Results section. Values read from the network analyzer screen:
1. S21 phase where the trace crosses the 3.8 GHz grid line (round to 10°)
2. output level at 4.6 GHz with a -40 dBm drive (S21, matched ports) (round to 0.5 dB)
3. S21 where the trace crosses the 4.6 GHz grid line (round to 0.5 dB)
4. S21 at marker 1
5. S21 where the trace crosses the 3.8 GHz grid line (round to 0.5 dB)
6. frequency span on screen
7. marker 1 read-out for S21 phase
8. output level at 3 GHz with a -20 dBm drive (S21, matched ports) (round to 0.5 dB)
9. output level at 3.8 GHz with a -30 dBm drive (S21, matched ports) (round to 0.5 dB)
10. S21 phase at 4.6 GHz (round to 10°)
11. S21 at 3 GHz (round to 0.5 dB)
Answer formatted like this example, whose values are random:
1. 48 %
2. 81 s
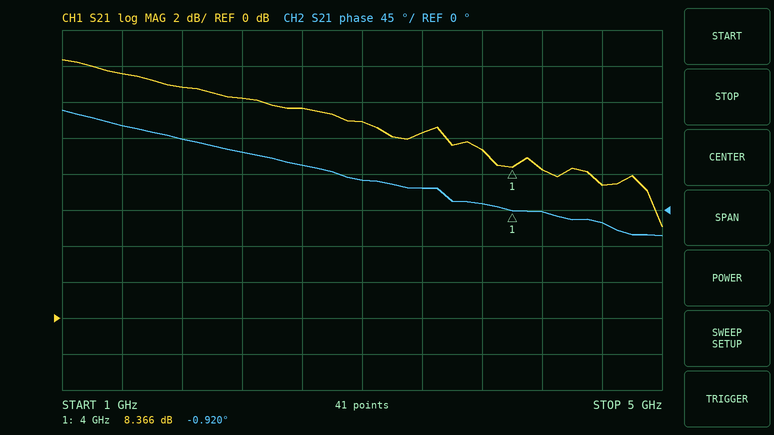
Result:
1. 10°
2. -32.5 dBm
3. 7.5 dB
4. 8.366 dB
5. 9.5 dB
6. 4 GHz
7. -0.920°
8. -9.0 dBm
9. -20.5 dBm
10. -20°
11. 11.0 dB
